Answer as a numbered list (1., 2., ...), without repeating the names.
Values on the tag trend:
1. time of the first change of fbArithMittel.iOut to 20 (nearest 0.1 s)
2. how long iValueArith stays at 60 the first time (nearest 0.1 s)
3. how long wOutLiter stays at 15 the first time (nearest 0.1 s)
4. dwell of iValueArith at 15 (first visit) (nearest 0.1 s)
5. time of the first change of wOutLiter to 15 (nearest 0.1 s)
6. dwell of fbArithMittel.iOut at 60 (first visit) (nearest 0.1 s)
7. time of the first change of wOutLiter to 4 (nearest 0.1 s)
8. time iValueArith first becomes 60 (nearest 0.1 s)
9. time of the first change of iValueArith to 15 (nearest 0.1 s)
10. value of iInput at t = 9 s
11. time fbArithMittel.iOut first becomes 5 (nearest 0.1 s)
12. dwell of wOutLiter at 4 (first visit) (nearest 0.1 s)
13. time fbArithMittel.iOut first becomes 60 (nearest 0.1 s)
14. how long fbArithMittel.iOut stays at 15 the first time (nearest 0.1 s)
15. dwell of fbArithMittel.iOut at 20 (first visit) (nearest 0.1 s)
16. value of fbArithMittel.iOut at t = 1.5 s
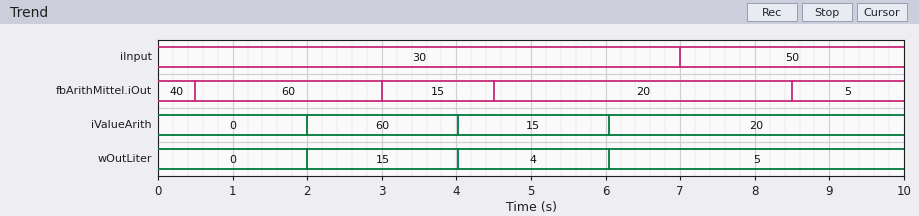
1. 4.5 s
2. 2.0 s
3. 2.0 s
4. 2.0 s
5. 2.0 s
6. 2.5 s
7. 4.0 s
8. 2.0 s
9. 4.0 s
10. 50
11. 8.5 s
12. 2.0 s
13. 0.5 s
14. 1.5 s
15. 4.0 s
16. 60
